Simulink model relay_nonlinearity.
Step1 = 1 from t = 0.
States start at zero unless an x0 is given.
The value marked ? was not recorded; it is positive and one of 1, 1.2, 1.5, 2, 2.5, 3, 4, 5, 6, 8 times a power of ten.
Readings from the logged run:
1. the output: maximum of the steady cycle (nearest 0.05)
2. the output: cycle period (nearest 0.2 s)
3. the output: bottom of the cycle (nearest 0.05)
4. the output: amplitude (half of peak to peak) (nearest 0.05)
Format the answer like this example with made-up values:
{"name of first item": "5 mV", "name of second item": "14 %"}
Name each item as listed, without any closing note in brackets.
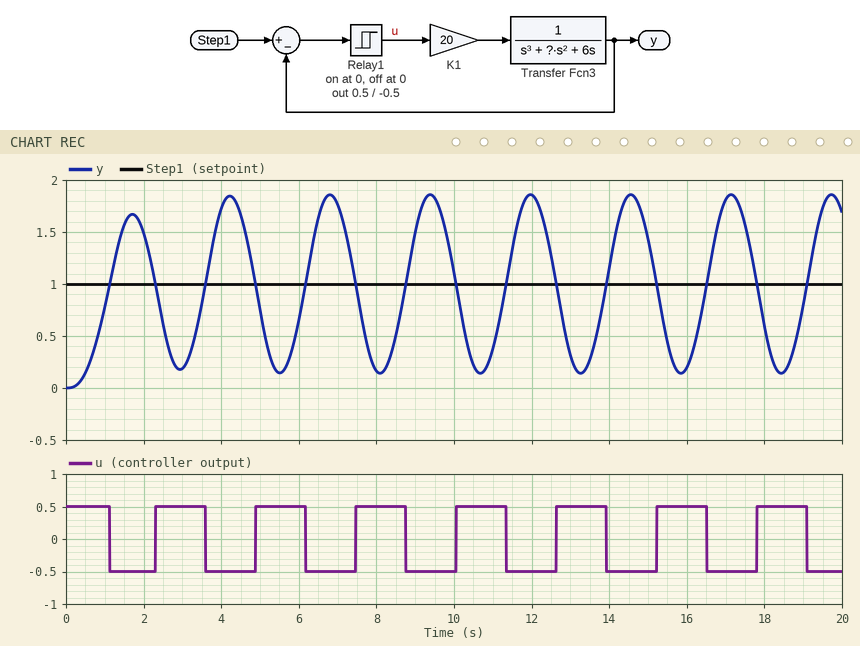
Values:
{"the output: maximum of the steady cycle": "1.85", "the output: cycle period": "2.6 s", "the output: bottom of the cycle": "0.15", "the output: amplitude (half of peak to peak)": "0.85"}
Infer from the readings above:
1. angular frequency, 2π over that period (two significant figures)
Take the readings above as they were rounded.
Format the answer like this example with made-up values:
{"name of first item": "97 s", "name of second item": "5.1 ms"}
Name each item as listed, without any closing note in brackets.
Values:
{"angular frequency, 2π over that period": "2.4 rad/s"}
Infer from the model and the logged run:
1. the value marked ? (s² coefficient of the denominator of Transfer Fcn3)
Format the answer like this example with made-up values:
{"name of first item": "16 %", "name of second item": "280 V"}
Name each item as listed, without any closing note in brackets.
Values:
{"the value marked ?": "2.5"}
